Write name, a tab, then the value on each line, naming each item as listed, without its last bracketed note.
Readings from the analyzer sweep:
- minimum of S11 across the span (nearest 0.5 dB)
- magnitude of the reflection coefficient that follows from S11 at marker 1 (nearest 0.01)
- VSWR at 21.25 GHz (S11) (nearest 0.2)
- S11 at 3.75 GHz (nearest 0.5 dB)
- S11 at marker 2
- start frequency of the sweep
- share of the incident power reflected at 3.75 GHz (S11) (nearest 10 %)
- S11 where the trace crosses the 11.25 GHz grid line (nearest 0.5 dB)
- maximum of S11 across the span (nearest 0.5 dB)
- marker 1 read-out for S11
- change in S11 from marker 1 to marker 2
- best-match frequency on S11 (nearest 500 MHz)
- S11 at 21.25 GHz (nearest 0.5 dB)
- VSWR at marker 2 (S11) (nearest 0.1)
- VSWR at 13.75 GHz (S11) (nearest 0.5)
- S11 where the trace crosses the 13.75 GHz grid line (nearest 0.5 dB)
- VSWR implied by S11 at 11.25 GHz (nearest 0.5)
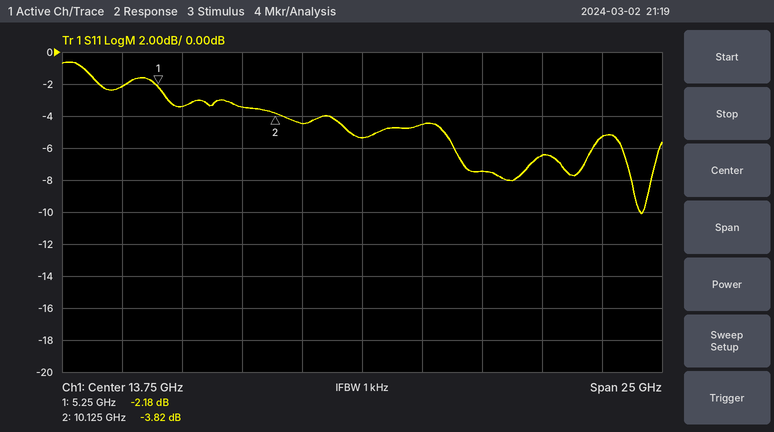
minimum of S11 across the span	-10.0 dB
magnitude of the reflection coefficient that follows from S11 at marker 1	0.78
VSWR at 21.25 GHz (S11)	2.8
S11 at 3.75 GHz	-2.0 dB
S11 at marker 2	-3.82 dB
start frequency of the sweep	1.25 GHz
share of the incident power reflected at 3.75 GHz (S11)	60 %
S11 where the trace crosses the 11.25 GHz grid line	-4.5 dB
maximum of S11 across the span	-0.5 dB
marker 1 read-out for S11	-2.18 dB
change in S11 from marker 1 to marker 2	-1.64 dB
best-match frequency on S11	25.5 GHz
S11 at 21.25 GHz	-6.5 dB
VSWR at marker 2 (S11)	4.6
VSWR at 13.75 GHz (S11)	3.5
S11 where the trace crosses the 13.75 GHz grid line	-5.5 dB
VSWR implied by S11 at 11.25 GHz	4.0
